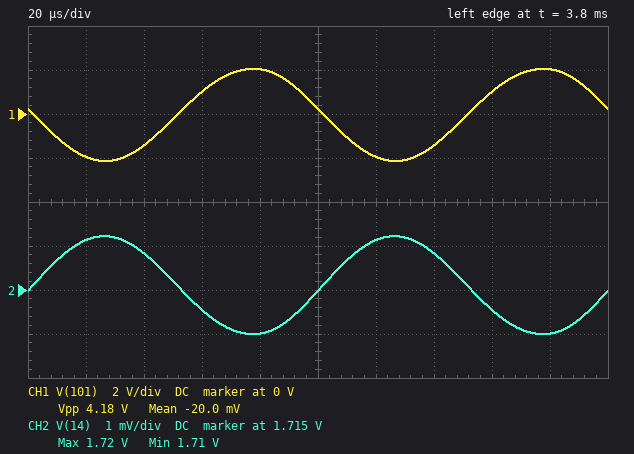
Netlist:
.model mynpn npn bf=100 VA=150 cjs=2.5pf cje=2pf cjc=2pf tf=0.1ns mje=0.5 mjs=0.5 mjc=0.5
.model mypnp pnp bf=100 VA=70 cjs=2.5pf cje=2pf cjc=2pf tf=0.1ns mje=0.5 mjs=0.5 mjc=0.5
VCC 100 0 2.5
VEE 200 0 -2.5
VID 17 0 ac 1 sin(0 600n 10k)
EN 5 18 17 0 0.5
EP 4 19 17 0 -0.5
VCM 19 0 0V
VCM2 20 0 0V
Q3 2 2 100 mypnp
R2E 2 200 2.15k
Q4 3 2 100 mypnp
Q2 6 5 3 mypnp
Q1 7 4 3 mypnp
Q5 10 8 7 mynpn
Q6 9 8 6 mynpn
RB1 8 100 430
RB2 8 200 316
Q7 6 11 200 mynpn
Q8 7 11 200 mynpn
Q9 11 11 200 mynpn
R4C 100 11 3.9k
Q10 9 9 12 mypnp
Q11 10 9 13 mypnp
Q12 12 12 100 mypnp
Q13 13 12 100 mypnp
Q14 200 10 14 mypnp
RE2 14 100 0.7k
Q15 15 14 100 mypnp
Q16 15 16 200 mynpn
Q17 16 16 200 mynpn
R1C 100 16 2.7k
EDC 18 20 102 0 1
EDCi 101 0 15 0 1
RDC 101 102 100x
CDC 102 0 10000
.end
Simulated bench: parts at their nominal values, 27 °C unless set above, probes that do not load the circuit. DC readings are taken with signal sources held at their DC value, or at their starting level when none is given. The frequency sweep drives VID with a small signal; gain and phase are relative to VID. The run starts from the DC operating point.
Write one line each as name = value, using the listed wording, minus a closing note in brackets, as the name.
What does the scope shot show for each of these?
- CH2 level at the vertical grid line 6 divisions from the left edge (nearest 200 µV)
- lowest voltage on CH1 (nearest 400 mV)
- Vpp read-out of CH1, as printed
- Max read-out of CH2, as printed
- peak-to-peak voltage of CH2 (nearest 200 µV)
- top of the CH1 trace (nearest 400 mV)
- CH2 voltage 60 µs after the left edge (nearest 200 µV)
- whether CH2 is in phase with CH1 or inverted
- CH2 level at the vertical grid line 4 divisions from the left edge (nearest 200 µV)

CH2 level at the vertical grid line 6 divisions from the left edge = 1.7162 V
lowest voltage on CH1 = -2.0 V
Vpp read-out of CH1, as printed = 4.18 V
Max read-out of CH2, as printed = 1.72 V
peak-to-peak voltage of CH2 = 2.2 mV
top of the CH1 trace = 2.0 V
CH2 voltage 60 µs after the left edge = 1.7146 V
whether CH2 is in phase with CH1 or inverted = inverted
CH2 level at the vertical grid line 4 divisions from the left edge = 1.7140 V
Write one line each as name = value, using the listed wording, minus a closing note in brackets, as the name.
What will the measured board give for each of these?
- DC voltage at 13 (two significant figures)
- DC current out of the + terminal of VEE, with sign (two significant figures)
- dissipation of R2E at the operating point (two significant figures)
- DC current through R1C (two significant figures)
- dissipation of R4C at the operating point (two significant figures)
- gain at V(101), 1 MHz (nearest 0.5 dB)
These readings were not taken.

DC voltage at 13 = 1.8 V
DC current out of the + terminal of VEE, with sign = -16 mA
dissipation of R2E at the operating point = 8.2 mW
DC current through R1C = 1.6 mA
dissipation of R4C at the operating point = 4.6 mW
gain at V(101), 1 MHz = 109.5 dB
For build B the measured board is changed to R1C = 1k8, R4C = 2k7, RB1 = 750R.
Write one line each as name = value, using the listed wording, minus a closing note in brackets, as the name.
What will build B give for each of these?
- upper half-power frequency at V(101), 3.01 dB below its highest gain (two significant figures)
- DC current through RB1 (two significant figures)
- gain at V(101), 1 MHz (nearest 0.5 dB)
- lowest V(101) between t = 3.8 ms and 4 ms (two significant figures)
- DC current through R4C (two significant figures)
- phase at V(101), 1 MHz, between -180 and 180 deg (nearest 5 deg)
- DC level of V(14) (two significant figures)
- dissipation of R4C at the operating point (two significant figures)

upper half-power frequency at V(101), 3.01 dB below its highest gain = 110 kHz
DC current through RB1 = 4.7 mA
gain at V(101), 1 MHz = 110.0 dB
lowest V(101) between t = 3.8 ms and 4 ms = -1.9 V
DC current through R4C = 1.6 mA
phase at V(101), 1 MHz, between -180 and 180 deg = 75 deg
DC level of V(14) = 1.7 V
dissipation of R4C at the operating point = 6.6 mW
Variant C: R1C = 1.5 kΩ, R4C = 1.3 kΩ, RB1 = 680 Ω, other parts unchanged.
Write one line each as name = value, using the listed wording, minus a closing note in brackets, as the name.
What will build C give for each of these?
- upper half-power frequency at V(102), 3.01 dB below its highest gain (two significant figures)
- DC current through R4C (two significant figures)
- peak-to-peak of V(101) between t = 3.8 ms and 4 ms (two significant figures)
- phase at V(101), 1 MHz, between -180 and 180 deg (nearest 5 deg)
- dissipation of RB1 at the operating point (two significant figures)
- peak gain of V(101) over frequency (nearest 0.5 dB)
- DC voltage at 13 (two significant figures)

upper half-power frequency at V(102), 3.01 dB below its highest gain = 440 mHz
DC current through R4C = 3.2 mA
peak-to-peak of V(101) between t = 3.8 ms and 4 ms = 3.3 V
phase at V(101), 1 MHz, between -180 and 180 deg = 75 deg
dissipation of RB1 at the operating point = 17 mW
peak gain of V(101) over frequency = 129.0 dB
DC voltage at 13 = 1.7 V
